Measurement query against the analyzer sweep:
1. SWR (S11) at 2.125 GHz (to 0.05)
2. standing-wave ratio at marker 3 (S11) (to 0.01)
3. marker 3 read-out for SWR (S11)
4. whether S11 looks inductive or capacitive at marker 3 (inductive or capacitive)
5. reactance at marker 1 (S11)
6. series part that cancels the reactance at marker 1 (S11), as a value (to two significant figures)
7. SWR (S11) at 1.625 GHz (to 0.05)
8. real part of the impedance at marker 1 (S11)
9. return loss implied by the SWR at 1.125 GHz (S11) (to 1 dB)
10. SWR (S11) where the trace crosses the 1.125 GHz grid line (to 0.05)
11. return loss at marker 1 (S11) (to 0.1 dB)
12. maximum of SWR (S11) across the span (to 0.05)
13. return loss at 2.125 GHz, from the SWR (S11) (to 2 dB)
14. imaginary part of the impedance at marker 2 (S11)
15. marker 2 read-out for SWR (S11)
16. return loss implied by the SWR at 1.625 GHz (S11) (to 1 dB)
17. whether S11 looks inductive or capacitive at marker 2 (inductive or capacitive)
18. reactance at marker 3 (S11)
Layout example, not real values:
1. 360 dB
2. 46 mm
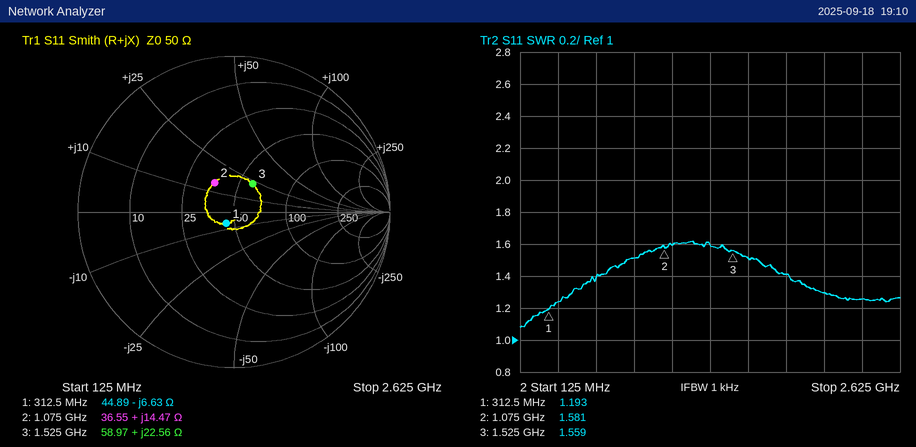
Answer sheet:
1. 1.30
2. 1.56
3. 1.559
4. inductive
5. -6.63 Ω
6. 3.4 nH
7. 1.50
8. 44.89 Ω
9. 13 dB
10. 1.60
11. 21.1 dB
12. 1.60
13. 18 dB
14. +14.47 Ω
15. 1.581
16. 14 dB
17. inductive
18. +22.56 Ω
